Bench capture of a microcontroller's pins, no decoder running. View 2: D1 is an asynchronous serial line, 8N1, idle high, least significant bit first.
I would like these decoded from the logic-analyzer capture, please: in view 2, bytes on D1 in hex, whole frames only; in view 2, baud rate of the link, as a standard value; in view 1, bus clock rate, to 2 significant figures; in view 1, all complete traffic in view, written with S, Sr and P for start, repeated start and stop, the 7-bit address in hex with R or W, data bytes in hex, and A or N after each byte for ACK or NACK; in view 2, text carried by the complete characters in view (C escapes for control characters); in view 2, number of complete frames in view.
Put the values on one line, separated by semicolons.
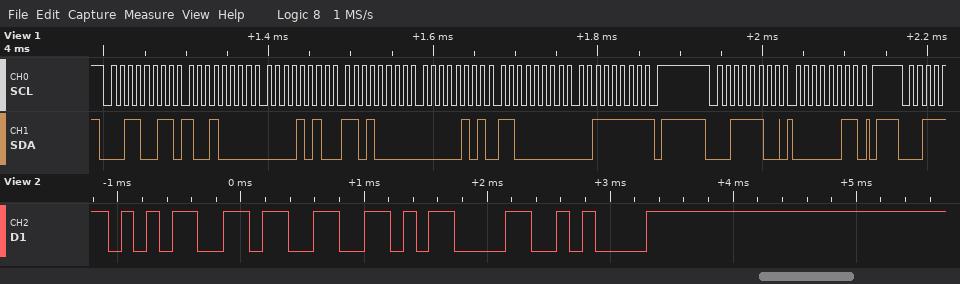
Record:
35 33 0D 0A; 9600 baud; 100 kHz; S 19R A 90 A 0A A D0 A 05 A C0 A 3F N P S 1EW A 03 A P; "53\r\n"; 4
